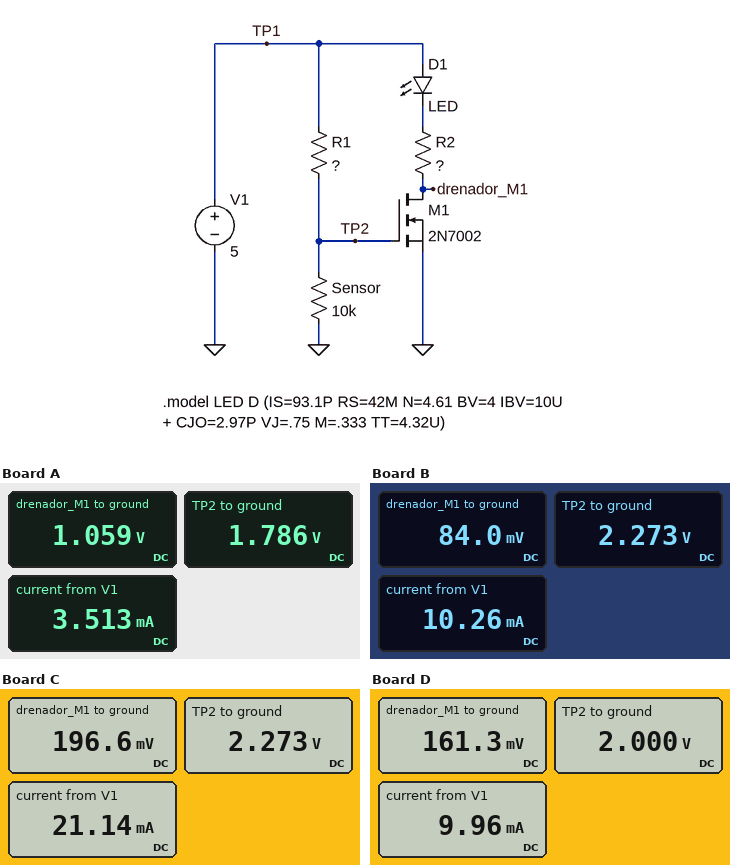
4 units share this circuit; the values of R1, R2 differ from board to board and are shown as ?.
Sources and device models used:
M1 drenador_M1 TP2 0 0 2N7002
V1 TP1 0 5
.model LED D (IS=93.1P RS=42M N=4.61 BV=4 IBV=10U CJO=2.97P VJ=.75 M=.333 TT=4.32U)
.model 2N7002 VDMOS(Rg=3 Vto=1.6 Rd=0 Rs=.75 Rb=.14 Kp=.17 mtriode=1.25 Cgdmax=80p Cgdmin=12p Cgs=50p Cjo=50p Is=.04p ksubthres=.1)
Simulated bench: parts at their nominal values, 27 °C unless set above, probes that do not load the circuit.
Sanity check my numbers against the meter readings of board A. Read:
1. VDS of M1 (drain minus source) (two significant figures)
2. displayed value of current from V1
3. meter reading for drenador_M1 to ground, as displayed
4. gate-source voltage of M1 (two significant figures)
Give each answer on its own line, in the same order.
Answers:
1.1 V
3.513 mA
1.059 V
1.8 V
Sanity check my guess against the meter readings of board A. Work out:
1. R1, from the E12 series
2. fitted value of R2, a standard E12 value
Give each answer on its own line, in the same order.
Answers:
18 kΩ
560 Ω
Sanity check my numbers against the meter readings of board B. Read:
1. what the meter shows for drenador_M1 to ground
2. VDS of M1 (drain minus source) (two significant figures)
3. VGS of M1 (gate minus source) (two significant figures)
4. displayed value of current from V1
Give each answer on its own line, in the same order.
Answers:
84.0 mV
84 mV
2.3 V
10.26 mA
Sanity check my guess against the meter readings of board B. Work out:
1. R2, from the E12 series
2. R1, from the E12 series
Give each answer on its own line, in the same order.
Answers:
270 Ω
12 kΩ
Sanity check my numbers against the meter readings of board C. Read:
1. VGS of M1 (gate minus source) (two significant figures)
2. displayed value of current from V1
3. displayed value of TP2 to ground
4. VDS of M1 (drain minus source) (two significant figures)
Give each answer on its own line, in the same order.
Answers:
2.3 V
21.14 mA
2.273 V
200 mV
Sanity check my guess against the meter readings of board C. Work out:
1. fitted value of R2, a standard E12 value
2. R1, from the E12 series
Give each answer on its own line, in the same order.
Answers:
120 Ω
12 kΩ
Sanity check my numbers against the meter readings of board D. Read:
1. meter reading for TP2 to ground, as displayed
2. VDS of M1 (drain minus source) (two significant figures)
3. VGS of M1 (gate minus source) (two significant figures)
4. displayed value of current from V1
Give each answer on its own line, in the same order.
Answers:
2.000 V
160 mV
2.0 V
9.96 mA
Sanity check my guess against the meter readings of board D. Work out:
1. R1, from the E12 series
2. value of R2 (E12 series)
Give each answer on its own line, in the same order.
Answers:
15 kΩ
270 Ω
